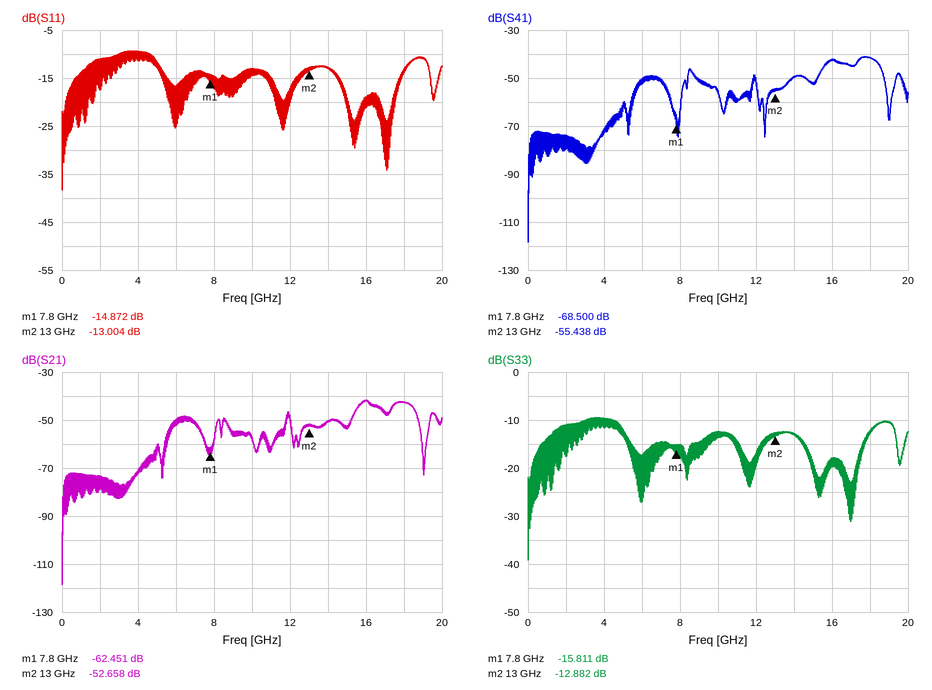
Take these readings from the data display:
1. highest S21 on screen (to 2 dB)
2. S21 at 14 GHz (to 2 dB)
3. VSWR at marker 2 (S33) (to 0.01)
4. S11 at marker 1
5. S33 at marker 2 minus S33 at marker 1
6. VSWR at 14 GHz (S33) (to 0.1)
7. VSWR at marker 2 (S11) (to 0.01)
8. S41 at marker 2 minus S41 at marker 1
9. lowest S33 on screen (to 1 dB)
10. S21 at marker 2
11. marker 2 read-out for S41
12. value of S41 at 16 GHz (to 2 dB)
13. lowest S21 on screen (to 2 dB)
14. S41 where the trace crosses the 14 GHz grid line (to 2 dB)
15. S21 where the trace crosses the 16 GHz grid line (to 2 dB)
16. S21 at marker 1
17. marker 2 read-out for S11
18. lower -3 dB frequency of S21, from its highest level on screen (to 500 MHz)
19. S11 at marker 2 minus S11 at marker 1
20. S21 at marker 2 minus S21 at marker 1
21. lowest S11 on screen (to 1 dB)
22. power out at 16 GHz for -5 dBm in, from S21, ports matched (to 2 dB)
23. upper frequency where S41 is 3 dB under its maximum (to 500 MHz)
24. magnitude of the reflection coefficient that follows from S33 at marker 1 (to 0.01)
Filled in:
-42 dB
-50 dB
1.59
-14.872 dB
2.929 dB
1.6
1.58
13.062 dB
-39 dB
-52.658 dB
-55.438 dB
-42 dB
-118 dB
-50 dB
-42 dB
-62.451 dB
-13.004 dB
15.5 GHz
1.868 dB
9.793 dB
-38 dB
-46 dBm
18.5 GHz
0.16
